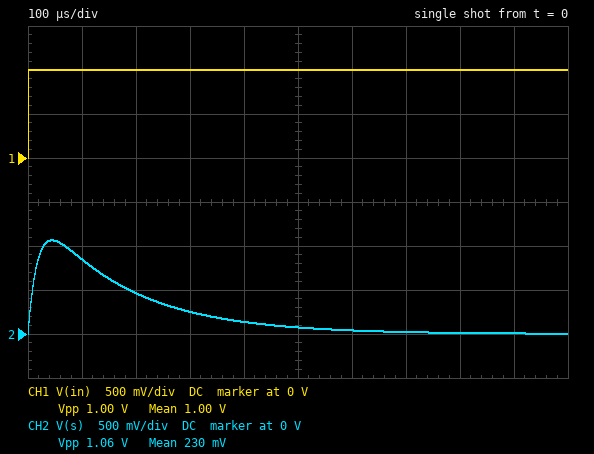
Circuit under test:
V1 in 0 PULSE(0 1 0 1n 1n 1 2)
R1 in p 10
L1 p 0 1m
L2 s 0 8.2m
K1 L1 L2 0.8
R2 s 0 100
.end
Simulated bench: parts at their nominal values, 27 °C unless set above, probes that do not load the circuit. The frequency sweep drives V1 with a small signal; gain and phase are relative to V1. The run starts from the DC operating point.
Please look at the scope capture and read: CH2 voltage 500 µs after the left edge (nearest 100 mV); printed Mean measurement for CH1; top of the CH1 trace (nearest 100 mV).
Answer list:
100 mV
1.00 V
1.0 V
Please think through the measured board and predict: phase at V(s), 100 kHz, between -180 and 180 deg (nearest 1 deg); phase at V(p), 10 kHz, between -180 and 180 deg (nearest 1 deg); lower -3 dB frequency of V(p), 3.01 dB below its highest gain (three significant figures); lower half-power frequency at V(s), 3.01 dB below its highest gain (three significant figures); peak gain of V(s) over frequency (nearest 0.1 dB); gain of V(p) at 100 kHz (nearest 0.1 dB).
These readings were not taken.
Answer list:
-84 deg
19 deg
4.90 kHz
808 Hz
2.0 dB
0 dB
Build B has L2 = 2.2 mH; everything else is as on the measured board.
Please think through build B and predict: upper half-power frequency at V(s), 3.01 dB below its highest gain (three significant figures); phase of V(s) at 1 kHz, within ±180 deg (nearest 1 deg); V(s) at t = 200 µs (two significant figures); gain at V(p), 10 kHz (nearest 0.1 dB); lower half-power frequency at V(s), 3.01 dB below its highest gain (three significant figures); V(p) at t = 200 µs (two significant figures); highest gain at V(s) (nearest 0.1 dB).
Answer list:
25.8 kHz
52 deg
190 mV
-1.1 dB
1.24 kHz
150 mV
-0.2 dB
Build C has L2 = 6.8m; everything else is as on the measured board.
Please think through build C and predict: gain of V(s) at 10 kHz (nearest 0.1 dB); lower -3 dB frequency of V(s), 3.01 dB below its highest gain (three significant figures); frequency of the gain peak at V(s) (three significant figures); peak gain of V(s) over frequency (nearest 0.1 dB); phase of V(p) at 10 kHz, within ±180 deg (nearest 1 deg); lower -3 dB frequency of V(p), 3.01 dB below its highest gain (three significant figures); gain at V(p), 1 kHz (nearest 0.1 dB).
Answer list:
-0.4 dB
877 Hz
3.22 kHz
1.9 dB
18 deg
4.42 kHz
-6.8 dB
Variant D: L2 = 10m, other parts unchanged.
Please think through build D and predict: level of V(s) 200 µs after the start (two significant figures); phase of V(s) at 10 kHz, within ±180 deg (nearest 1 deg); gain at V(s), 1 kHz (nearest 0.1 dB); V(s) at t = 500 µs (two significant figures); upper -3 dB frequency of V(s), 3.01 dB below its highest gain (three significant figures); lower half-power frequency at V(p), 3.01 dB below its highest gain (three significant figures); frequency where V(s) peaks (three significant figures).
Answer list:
520 mV
-46 deg
0.4 dB
98 mV
9.58 kHz
5.18 kHz
2.65 kHz
